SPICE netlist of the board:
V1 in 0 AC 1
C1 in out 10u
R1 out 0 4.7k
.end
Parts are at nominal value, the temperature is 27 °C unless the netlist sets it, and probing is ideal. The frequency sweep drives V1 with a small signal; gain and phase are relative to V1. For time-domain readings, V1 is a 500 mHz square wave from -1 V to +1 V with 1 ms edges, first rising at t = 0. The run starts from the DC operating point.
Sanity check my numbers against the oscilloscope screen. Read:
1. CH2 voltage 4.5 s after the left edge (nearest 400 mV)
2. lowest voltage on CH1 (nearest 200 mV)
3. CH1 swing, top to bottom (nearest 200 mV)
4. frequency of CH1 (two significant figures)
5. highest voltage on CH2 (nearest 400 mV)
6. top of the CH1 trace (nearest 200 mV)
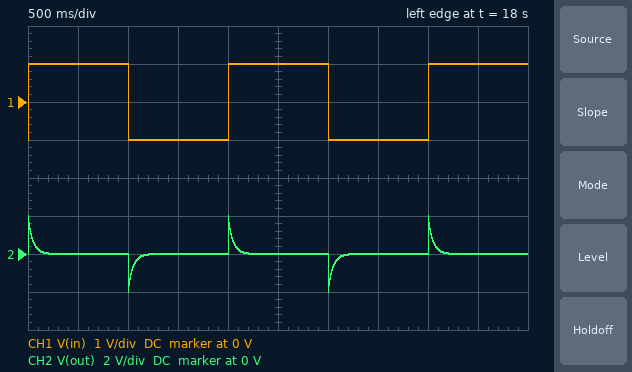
0 V
-1.0 V
2.0 V
500 mHz
2.0 V
1.0 V
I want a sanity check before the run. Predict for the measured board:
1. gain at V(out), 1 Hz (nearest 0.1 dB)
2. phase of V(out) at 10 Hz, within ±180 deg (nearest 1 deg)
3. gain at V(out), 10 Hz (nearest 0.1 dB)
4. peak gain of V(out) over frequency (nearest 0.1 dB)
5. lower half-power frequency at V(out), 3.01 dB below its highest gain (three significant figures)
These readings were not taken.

-11.0 dB
19 deg
-0.5 dB
0 dB
3.39 Hz
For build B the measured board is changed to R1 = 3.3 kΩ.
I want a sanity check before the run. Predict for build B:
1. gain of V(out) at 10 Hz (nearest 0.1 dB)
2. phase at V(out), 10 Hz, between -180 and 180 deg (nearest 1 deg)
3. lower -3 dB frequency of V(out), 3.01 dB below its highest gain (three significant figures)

-0.9 dB
26 deg
4.82 Hz
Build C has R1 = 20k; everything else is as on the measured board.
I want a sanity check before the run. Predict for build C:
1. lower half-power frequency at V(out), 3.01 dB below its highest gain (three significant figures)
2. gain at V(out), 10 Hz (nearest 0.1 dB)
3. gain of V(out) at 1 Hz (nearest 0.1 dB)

796 mHz
0 dB
-2.1 dB
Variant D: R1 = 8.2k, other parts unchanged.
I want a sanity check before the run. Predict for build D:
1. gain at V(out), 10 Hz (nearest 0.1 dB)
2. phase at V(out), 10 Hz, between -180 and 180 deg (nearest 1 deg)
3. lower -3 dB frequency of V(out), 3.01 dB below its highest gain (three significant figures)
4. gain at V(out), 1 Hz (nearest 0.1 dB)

-0.2 dB
11 deg
1.94 Hz
-6.8 dB
